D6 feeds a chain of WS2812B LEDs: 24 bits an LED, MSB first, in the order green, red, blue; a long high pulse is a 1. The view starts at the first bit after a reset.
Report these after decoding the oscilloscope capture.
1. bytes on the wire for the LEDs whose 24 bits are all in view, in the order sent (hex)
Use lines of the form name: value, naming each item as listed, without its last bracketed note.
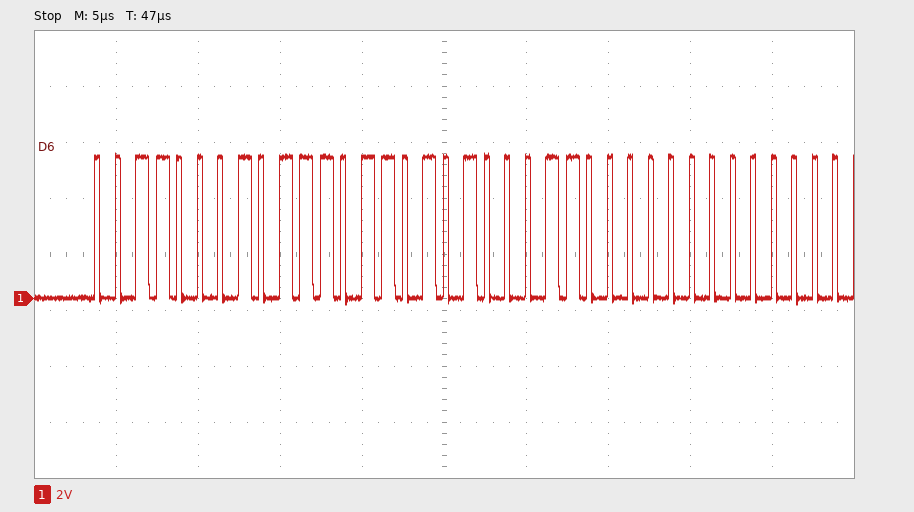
bytes on the wire for the LEDs whose 24 bits are all in view, in the order sent: 31 76 A3
